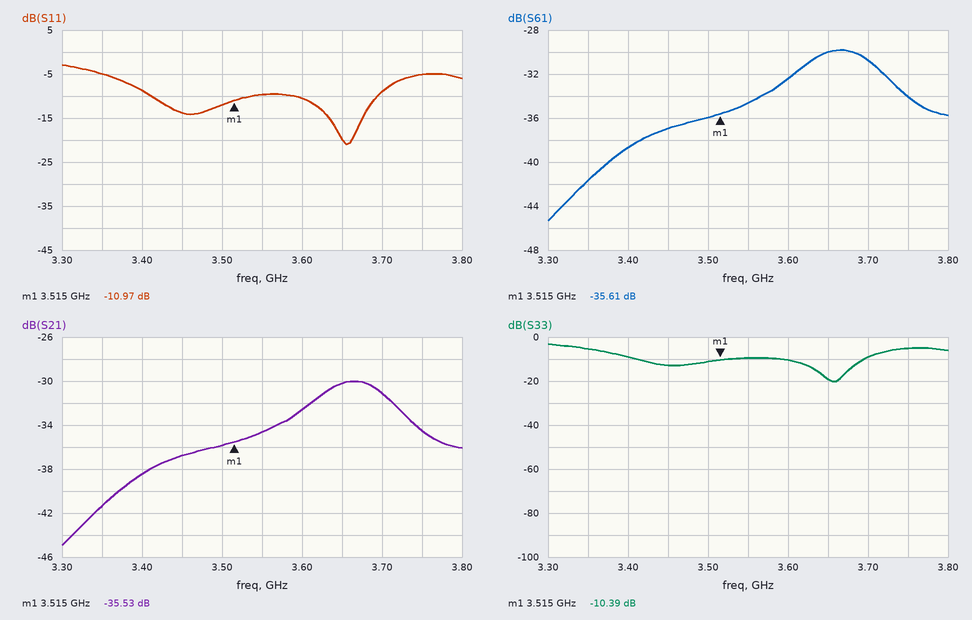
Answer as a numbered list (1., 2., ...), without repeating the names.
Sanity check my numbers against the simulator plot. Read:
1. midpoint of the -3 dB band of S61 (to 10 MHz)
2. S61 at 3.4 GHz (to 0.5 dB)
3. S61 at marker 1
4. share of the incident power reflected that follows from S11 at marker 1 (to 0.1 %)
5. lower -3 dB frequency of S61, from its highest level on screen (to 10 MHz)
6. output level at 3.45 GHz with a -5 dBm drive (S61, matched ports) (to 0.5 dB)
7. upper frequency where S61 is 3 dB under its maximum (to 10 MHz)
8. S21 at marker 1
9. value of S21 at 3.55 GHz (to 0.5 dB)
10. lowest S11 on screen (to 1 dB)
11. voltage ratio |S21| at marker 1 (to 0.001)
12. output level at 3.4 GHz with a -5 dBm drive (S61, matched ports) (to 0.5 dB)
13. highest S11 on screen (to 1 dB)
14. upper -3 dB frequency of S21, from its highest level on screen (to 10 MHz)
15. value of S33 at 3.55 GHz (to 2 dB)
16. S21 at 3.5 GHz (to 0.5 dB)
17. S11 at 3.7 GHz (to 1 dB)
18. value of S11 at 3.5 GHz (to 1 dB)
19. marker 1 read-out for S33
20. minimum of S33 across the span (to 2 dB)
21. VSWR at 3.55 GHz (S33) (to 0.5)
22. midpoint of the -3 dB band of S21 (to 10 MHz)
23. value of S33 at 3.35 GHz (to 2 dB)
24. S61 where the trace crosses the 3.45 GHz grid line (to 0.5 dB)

1. 3.66 GHz
2. -38.5 dB
3. -35.61 dB
4. 8.0 %
5. 3.59 GHz
6. -42.0 dBm
7. 3.73 GHz
8. -35.53 dB
9. -34.5 dB
10. -21 dB
11. 0.017
12. -43.5 dBm
13. -3 dB
14. 3.73 GHz
15. -10 dB
16. -36.0 dB
17. -9 dB
18. -12 dB
19. -10.39 dB
20. -20 dB
21. 2.0
22. 3.66 GHz
23. -6 dB
24. -37.0 dB
